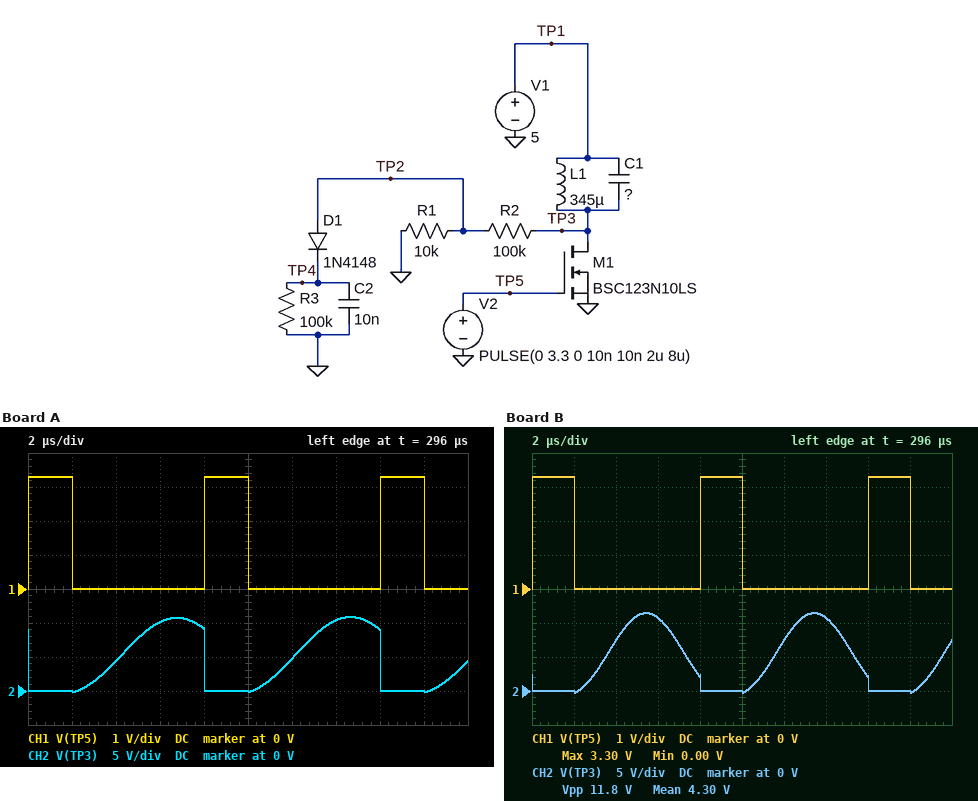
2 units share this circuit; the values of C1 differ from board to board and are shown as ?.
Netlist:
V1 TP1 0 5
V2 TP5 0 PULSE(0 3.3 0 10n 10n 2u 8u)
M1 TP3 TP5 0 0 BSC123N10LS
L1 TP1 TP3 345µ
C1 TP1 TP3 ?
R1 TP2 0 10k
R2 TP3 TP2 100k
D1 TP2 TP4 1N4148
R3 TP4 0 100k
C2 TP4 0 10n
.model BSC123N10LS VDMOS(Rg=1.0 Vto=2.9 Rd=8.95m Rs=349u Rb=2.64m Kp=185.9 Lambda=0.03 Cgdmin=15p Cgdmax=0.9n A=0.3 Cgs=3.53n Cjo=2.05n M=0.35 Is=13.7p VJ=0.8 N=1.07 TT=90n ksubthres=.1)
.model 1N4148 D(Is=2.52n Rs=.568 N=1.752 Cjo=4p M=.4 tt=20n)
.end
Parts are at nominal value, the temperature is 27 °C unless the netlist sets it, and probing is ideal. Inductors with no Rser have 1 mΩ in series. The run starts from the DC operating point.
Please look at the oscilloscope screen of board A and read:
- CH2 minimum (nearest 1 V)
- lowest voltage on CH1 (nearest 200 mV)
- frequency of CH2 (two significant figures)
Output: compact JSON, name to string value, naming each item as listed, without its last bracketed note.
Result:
{"CH2 minimum": "0 V", "lowest voltage on CH1": "0 V", "frequency of CH2": "130 kHz"}
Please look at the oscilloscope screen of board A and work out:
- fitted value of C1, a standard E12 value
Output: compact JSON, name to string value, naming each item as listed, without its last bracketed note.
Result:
{"fitted value of C1, a standard E12 value": "6.8 nF"}
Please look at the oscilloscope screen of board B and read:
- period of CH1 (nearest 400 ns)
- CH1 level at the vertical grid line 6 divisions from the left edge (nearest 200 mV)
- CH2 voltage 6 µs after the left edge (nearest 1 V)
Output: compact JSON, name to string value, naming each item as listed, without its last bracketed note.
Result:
{"period of CH1": "8.0 µs", "CH1 level at the vertical grid line 6 divisions from the left edge": "0 V", "CH2 voltage 6 µs after the left edge": "11 V"}
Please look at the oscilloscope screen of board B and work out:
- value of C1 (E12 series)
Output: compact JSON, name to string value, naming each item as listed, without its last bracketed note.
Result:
{"value of C1": "3.3 nF"}
